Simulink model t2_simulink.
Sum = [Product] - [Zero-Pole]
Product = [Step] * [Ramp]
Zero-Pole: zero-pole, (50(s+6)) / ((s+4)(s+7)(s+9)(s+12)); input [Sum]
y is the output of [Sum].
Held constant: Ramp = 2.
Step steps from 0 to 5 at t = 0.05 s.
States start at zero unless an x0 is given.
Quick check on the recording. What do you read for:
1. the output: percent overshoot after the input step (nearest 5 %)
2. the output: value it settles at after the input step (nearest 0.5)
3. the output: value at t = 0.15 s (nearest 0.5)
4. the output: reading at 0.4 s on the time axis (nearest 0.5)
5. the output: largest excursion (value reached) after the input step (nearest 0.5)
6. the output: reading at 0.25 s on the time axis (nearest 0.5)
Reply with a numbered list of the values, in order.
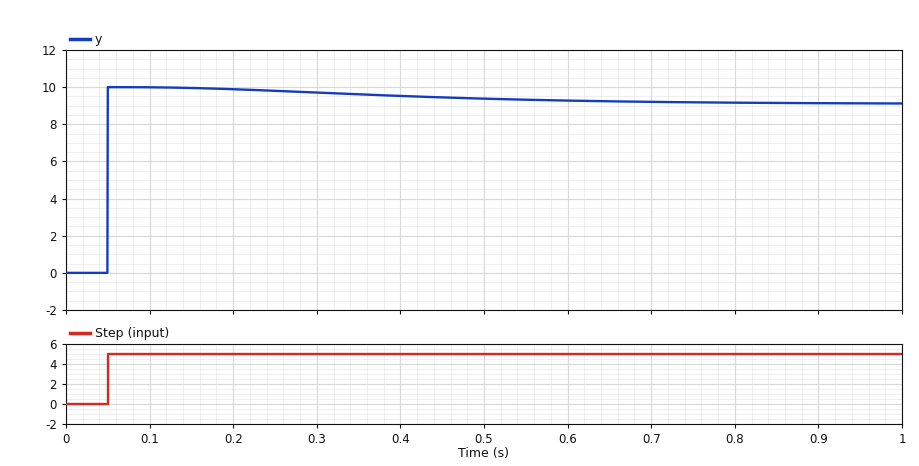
1. 10 %
2. 9.0
3. 10.0
4. 9.5
5. 10.0
6. 10.0
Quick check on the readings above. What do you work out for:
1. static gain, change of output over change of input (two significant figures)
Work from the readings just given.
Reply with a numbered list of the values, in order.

1. 1.8
